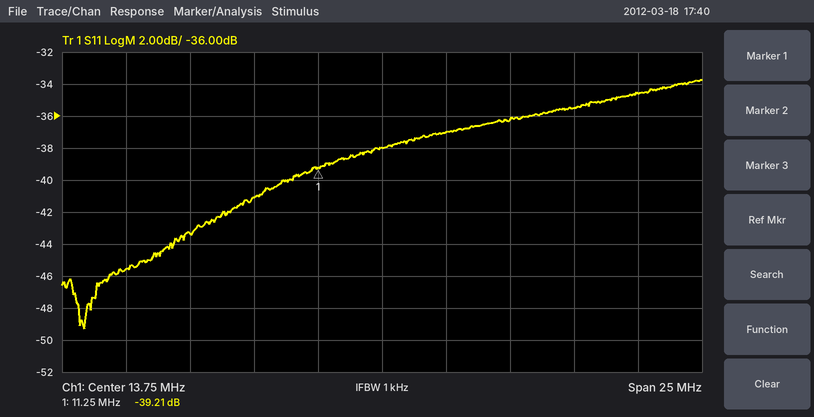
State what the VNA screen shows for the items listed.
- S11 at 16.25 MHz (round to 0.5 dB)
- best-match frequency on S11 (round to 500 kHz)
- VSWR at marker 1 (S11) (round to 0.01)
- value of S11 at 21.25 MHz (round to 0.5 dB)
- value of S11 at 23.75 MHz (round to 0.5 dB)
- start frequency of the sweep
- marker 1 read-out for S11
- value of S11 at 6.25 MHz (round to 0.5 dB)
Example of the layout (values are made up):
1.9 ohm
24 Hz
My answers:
-37.0 dB
2.0 MHz
1.02
-35.5 dB
-34.5 dB
1.25 MHz
-39.21 dB
-43.5 dB
